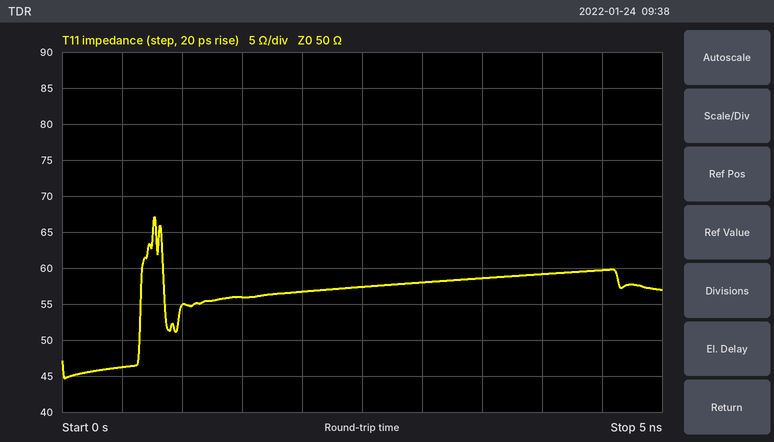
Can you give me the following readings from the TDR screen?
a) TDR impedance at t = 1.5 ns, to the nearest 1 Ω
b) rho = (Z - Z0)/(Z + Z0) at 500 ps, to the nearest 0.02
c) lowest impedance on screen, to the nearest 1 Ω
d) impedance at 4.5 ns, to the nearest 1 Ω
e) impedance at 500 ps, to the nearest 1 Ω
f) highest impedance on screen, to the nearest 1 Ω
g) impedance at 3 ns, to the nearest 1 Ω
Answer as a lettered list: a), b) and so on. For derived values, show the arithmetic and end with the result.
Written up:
a) 56 Ω
b) (46 − 50)/(46 + 50) ≈ -0.04
c) 45 Ω
d) 60 Ω
e) 46 Ω
f) 67 Ω
g) 58 Ω
